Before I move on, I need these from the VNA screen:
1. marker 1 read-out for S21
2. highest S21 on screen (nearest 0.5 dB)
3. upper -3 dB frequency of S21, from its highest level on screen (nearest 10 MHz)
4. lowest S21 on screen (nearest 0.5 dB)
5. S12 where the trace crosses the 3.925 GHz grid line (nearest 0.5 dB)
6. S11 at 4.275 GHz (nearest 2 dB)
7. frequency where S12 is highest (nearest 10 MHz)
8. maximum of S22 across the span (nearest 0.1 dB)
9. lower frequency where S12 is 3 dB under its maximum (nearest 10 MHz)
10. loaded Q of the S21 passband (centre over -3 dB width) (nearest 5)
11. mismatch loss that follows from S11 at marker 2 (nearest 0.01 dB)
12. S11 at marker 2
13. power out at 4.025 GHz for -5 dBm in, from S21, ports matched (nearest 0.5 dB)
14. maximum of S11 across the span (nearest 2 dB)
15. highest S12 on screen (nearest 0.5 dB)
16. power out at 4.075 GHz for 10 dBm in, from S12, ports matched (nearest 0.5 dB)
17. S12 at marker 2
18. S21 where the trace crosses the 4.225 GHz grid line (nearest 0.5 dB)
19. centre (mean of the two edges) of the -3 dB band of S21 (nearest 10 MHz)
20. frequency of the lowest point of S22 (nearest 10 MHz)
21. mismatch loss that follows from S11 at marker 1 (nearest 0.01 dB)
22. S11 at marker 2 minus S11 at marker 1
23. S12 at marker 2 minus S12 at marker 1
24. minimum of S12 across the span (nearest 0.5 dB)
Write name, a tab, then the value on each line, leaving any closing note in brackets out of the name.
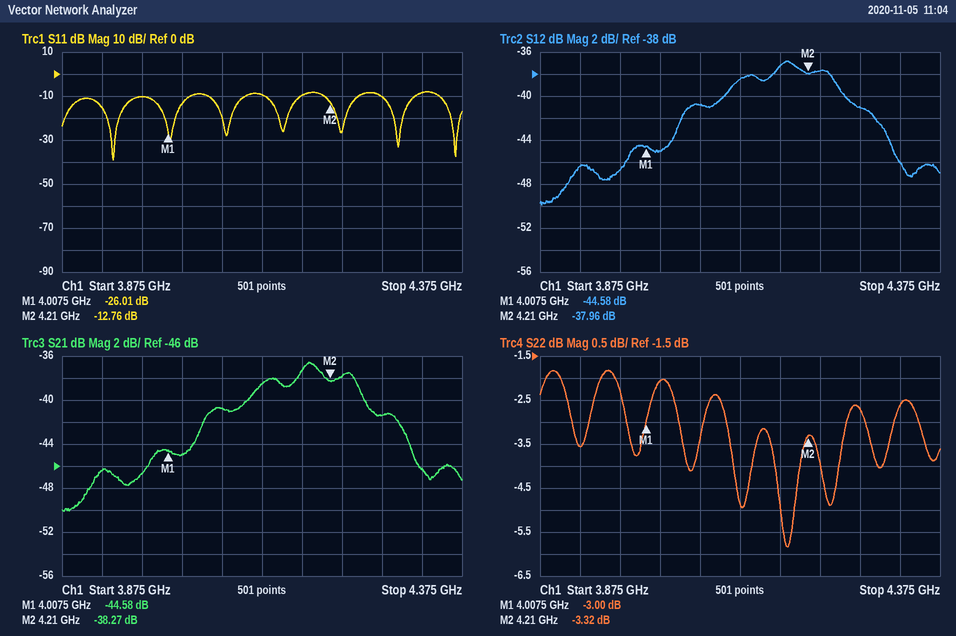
marker 1 read-out for S21	-44.58 dB
highest S21 on screen	-36.5 dB
upper -3 dB frequency of S21, from its highest level on screen	4.25 GHz
lowest S21 on screen	-50.0 dB
S12 where the trace crosses the 3.925 GHz grid line	-46.5 dB
S11 at 4.275 GHz	-10 dB
frequency where S12 is highest	4.18 GHz
maximum of S22 across the span	-1.8 dB
lower frequency where S12 is 3 dB under its maximum	4.11 GHz
loaded Q of the S21 passband (centre over -3 dB width)	30
mismatch loss that follows from S11 at marker 2	0.24 dB
S11 at marker 2	-12.76 dB
power out at 4.025 GHz for -5 dBm in, from S21, ports matched	-50.0 dBm
maximum of S11 across the span	-8 dB
highest S12 on screen	-37.0 dB
power out at 4.075 GHz for 10 dBm in, from S12, ports matched	-31.0 dBm
S12 at marker 2	-37.96 dB
S21 where the trace crosses the 4.225 GHz grid line	-38.0 dB
centre (mean of the two edges) of the -3 dB band of S21	4.18 GHz
frequency of the lowest point of S22	4.18 GHz
mismatch loss that follows from S11 at marker 1	0.01 dB
S11 at marker 2 minus S11 at marker 1	13.25 dB
S12 at marker 2 minus S12 at marker 1	6.62 dB
minimum of S12 across the span	-50.0 dB
